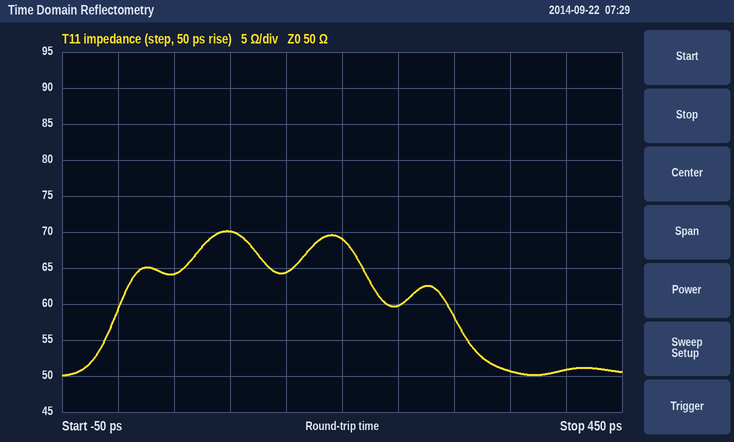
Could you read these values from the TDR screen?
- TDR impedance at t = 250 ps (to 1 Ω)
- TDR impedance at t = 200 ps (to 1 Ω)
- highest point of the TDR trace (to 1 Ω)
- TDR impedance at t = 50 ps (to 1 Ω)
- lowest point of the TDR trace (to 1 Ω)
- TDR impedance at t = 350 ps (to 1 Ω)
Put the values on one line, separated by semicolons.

60 Ω; 69 Ω; 70 Ω; 64 Ω; 50 Ω; 51 Ω
